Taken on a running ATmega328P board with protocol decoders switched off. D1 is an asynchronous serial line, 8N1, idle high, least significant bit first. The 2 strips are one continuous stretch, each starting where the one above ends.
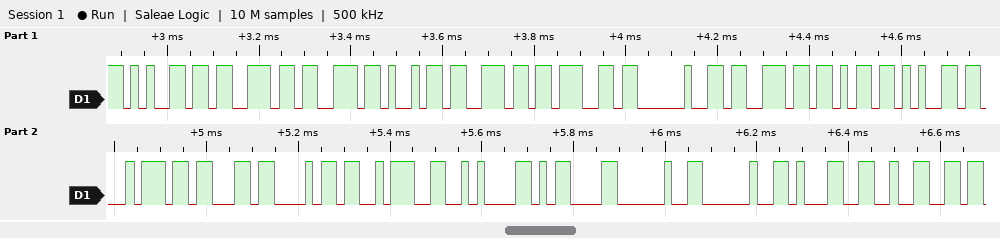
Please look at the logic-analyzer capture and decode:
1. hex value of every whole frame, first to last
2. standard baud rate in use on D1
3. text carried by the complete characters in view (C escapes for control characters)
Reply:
65 73 73 69 6E 67 20 73 6B 65 74 63 68 3A 0A 0D 20 20 31 32
57600 baud
"essing sketch:\n\r  12"
